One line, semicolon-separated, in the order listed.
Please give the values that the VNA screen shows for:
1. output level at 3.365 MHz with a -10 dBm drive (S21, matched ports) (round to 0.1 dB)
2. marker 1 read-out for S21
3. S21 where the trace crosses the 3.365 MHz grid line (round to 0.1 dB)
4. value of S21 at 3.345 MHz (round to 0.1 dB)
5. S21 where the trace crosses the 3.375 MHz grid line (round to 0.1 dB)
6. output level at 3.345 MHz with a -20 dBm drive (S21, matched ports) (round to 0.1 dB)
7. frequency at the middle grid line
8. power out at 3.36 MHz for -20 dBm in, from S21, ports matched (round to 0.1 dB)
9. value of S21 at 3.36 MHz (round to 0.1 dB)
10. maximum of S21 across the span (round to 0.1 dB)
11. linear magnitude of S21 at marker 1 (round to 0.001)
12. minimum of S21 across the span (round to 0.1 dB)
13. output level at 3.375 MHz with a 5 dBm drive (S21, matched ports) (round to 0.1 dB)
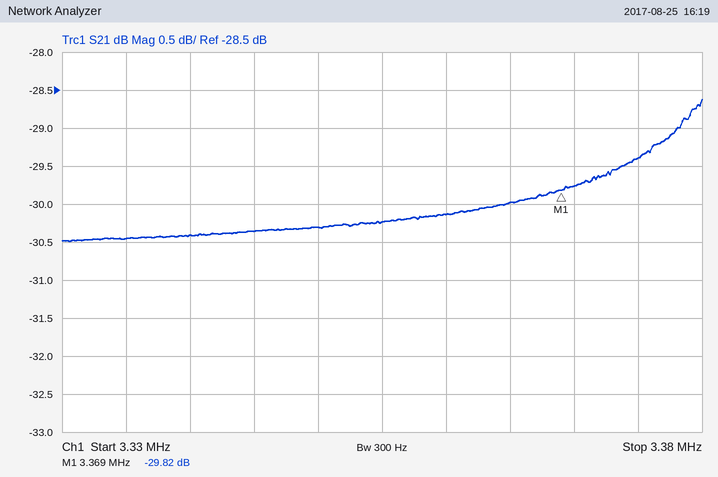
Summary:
-40.0 dBm; -29.82 dB; -30.0 dB; -30.4 dB; -29.4 dB; -50.4 dBm; 3.355 MHz; -50.1 dBm; -30.1 dB; -28.6 dB; 0.032; -30.5 dB; -24.4 dBm
